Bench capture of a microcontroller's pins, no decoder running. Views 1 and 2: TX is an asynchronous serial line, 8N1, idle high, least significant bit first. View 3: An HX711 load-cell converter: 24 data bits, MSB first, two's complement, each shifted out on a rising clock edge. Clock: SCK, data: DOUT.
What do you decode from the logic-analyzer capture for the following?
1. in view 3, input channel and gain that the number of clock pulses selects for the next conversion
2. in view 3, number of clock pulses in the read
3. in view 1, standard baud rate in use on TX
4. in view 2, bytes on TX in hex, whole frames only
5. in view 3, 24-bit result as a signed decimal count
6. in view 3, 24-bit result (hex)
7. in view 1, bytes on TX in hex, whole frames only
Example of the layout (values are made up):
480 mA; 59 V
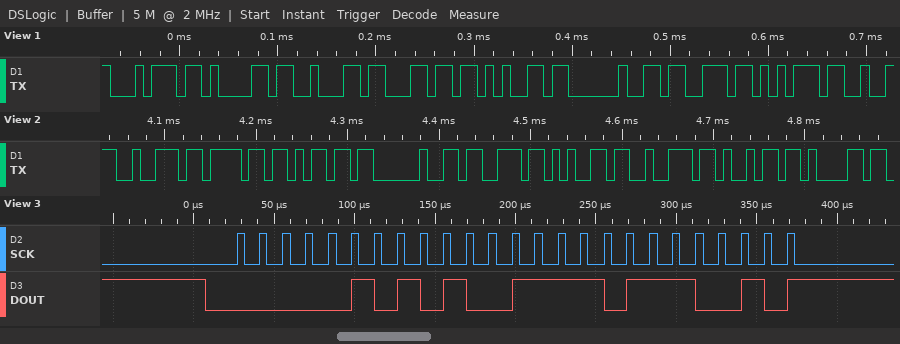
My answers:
channel A, gain 128; 25; 115200 baud; 72 6F 6D 20 73 65 72 69 61; 348018; 0x054F72; 0x74 0x61 0x62 0x6C 0x65 0x20 0x73 0x75
